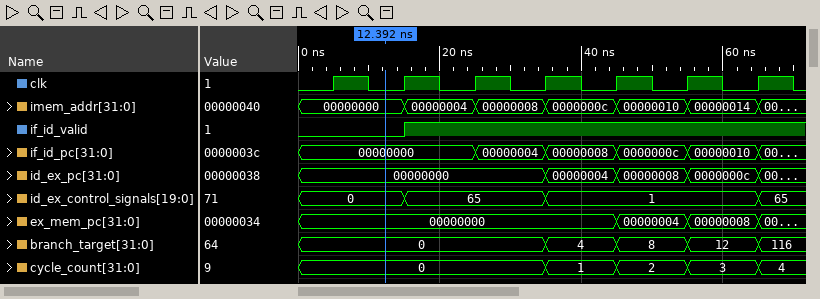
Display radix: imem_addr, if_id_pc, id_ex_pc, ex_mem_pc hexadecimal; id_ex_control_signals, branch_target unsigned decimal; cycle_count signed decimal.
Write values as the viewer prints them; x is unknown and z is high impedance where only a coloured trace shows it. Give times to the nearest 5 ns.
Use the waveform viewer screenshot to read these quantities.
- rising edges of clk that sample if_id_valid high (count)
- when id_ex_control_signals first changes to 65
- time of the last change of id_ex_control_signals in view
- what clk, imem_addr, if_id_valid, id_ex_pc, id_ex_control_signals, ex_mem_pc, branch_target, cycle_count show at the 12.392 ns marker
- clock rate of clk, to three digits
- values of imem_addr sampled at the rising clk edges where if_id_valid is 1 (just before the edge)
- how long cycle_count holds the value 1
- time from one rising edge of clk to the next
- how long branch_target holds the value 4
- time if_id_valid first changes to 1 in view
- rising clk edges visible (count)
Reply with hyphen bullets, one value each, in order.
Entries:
- 5
- 15 ns
- 65 ns
- clk=0, imem_addr=00000000, if_id_valid=0, id_ex_pc=00000000, id_ex_control_signals=0, ex_mem_pc=00000000, branch_target=0, cycle_count=0
- 100 MHz
- 00000004, 00000008, 0000000c, 00000010, 00000014
- 10 ns
- 10 ns
- 10 ns
- 15 ns
- 7
